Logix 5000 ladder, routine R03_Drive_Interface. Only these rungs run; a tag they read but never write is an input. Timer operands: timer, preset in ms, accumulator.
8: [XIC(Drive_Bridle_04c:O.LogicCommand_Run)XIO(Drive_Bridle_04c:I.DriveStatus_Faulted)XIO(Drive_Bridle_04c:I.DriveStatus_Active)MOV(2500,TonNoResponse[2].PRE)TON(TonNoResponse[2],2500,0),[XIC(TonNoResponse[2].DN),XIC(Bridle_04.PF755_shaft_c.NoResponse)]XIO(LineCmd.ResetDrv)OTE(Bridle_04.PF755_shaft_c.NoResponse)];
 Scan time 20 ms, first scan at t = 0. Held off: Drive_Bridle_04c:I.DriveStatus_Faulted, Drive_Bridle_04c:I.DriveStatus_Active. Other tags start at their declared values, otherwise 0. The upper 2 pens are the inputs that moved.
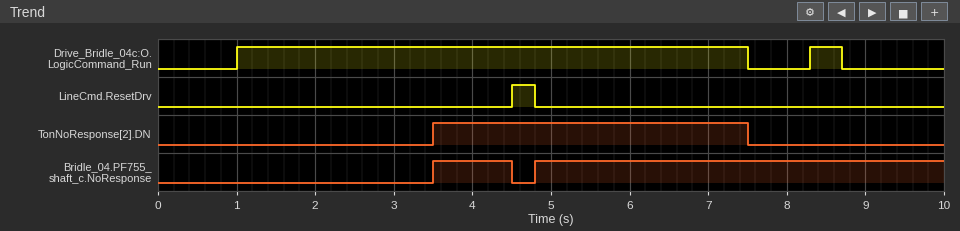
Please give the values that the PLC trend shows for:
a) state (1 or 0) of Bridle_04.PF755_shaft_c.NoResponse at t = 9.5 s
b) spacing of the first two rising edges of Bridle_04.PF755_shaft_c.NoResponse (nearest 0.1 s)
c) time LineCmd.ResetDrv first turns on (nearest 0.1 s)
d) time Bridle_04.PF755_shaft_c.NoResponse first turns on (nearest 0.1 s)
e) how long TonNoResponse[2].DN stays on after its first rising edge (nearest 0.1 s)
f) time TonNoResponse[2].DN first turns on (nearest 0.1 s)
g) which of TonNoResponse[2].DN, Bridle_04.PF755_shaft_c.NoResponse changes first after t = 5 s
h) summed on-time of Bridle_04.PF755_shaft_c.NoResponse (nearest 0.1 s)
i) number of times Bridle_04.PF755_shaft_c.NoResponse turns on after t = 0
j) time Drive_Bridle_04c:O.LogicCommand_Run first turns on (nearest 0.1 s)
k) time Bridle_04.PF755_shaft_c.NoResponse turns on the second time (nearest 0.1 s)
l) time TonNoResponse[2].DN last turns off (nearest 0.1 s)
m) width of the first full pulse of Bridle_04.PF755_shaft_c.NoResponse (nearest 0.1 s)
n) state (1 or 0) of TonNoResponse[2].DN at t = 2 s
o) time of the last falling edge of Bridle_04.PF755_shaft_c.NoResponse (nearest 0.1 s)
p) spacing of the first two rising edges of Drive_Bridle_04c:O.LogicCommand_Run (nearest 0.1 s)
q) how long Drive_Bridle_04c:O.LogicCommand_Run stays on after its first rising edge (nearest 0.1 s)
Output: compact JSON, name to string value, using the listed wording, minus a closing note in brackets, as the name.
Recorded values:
{"state (1 or 0) of Bridle_04.PF755_shaft_c.NoResponse at t = 9.5 s": "1", "spacing of the first two rising edges of Bridle_04.PF755_shaft_c.NoResponse": "1.3 s", "time LineCmd.ResetDrv first turns on": "4.5 s", "time Bridle_04.PF755_shaft_c.NoResponse first turns on": "3.5 s", "how long TonNoResponse[2].DN stays on after its first rising edge": "4.0 s", "time TonNoResponse[2].DN first turns on": "3.5 s", "which of TonNoResponse[2].DN, Bridle_04.PF755_shaft_c.NoResponse changes first after t = 5 s": "TonNoResponse[2].DN", "summed on-time of Bridle_04.PF755_shaft_c.NoResponse": "6.2 s", "number of times Bridle_04.PF755_shaft_c.NoResponse turns on after t = 0": "2", "time Drive_Bridle_04c:O.LogicCommand_Run first turns on": "1.0 s", "time Bridle_04.PF755_shaft_c.NoResponse turns on the second time": "4.8 s", "time TonNoResponse[2].DN last turns off": "7.5 s", "width of the first full pulse of Bridle_04.PF755_shaft_c.NoResponse": "1.0 s", "state (1 or 0) of TonNoResponse[2].DN at t = 2 s": "0", "time of the last falling edge of Bridle_04.PF755_shaft_c.NoResponse": "4.5 s", "spacing of the first two rising edges of Drive_Bridle_04c:O.LogicCommand_Run": "7.3 s", "how long Drive_Bridle_04c:O.LogicCommand_Run stays on after its first rising edge": "6.5 s"}
